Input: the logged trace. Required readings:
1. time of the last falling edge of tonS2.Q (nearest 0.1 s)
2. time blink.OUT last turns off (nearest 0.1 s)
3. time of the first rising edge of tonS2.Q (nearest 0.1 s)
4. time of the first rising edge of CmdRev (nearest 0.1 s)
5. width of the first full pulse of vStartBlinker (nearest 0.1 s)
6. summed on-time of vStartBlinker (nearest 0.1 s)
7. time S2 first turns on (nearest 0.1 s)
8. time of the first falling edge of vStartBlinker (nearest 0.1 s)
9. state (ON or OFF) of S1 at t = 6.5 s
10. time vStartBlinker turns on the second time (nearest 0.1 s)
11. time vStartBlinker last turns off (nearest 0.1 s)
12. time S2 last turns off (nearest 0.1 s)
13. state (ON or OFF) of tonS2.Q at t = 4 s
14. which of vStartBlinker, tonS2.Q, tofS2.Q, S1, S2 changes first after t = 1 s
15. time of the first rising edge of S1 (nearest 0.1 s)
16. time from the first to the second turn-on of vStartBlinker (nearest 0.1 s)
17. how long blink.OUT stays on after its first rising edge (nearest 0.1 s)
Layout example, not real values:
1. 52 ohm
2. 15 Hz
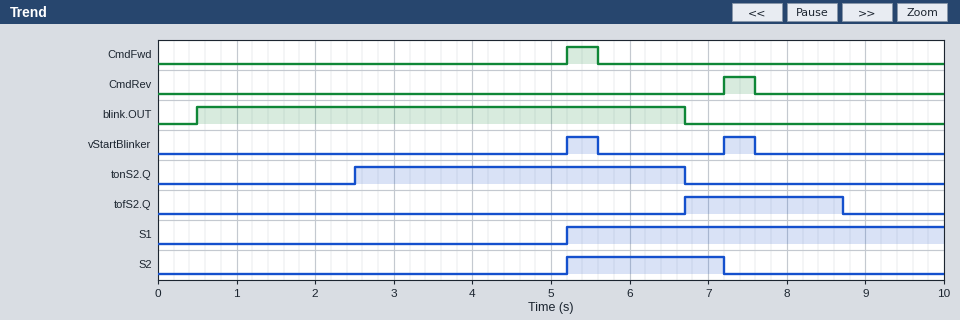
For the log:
1. 6.7 s
2. 6.7 s
3. 2.5 s
4. 7.2 s
5. 0.4 s
6. 0.8 s
7. 5.2 s
8. 5.6 s
9. ON
10. 7.2 s
11. 7.6 s
12. 7.2 s
13. ON
14. tonS2.Q
15. 5.2 s
16. 2.0 s
17. 6.2 s
